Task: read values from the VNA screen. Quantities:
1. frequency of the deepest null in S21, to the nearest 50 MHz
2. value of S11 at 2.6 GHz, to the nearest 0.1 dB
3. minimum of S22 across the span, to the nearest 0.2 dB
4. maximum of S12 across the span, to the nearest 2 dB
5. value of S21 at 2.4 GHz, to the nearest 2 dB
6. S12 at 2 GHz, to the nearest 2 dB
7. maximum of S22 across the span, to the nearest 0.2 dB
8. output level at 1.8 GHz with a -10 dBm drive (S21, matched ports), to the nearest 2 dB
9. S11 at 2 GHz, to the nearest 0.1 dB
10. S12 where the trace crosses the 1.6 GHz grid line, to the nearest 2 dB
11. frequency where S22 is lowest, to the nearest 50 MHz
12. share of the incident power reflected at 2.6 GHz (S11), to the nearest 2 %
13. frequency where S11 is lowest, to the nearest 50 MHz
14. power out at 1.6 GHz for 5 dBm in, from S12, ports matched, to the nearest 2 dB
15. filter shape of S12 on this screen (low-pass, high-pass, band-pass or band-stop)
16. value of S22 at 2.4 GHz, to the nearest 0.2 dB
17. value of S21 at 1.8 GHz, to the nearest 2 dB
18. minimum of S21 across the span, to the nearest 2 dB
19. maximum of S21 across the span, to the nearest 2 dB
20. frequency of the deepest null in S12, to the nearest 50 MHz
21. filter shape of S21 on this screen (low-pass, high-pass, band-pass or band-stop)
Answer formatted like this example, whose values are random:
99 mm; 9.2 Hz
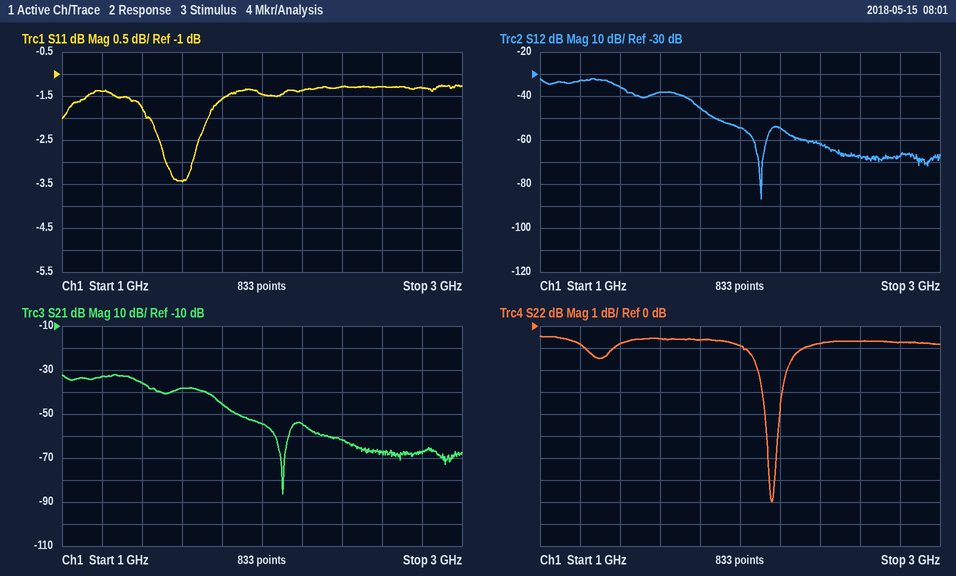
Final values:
2.10 GHz; -1.3 dB; -8.0 dB; -32 dB; -62 dB; -54 dB; -0.4 dB; -56 dBm; -1.5 dB; -38 dB; 2.15 GHz; 74 %; 1.60 GHz; -34 dBm; low-pass; -0.8 dB; -46 dB; -86 dB; -32 dB; 2.10 GHz; low-pass
